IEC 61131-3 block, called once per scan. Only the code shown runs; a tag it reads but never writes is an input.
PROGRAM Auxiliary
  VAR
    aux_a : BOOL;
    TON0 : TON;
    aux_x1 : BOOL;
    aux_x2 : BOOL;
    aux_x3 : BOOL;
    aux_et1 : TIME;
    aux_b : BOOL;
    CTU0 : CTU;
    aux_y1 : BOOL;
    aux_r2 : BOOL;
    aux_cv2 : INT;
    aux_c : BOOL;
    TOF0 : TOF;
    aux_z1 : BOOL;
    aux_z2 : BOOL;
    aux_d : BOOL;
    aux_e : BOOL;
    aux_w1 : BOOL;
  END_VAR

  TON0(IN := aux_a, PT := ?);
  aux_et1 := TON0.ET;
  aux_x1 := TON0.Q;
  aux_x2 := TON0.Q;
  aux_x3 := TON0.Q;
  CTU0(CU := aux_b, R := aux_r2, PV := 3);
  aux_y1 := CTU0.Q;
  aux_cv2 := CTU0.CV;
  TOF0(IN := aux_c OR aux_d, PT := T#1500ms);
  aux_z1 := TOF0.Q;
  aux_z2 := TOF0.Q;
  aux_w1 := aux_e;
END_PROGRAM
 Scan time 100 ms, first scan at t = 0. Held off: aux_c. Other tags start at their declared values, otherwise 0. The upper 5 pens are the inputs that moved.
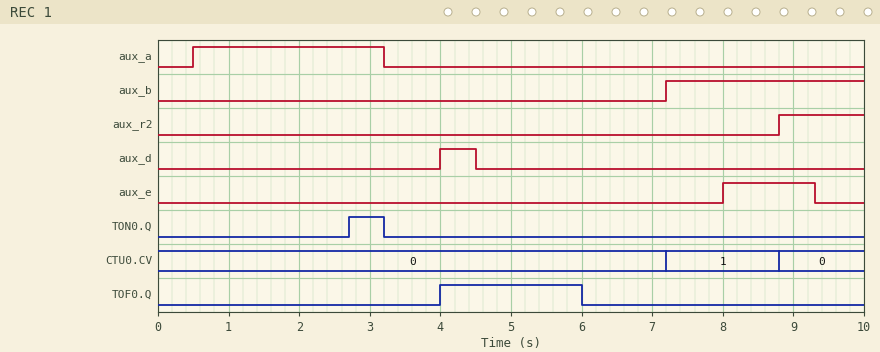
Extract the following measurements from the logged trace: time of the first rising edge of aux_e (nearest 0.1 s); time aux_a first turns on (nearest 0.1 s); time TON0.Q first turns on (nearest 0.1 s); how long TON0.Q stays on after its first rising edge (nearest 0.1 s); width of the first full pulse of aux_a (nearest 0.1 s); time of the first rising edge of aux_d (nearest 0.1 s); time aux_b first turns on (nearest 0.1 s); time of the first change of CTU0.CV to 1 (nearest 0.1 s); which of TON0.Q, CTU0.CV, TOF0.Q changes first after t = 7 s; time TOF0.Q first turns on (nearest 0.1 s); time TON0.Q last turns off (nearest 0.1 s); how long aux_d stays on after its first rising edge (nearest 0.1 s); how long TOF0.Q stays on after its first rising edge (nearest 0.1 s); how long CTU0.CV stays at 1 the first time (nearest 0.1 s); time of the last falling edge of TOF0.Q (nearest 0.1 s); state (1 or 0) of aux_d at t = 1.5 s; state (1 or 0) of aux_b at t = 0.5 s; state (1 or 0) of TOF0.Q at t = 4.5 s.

8.0 s
0.5 s
2.7 s
0.5 s
2.7 s
4.0 s
7.2 s
7.2 s
CTU0.CV
4.0 s
3.2 s
0.5 s
2.0 s
1.6 s
6.0 s
0
0
1
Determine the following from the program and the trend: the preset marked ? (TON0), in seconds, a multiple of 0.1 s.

2.2 s
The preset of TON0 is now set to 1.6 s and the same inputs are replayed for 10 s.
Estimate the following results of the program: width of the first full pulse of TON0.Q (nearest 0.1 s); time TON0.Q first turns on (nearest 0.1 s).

1.1 s
2.1 s
